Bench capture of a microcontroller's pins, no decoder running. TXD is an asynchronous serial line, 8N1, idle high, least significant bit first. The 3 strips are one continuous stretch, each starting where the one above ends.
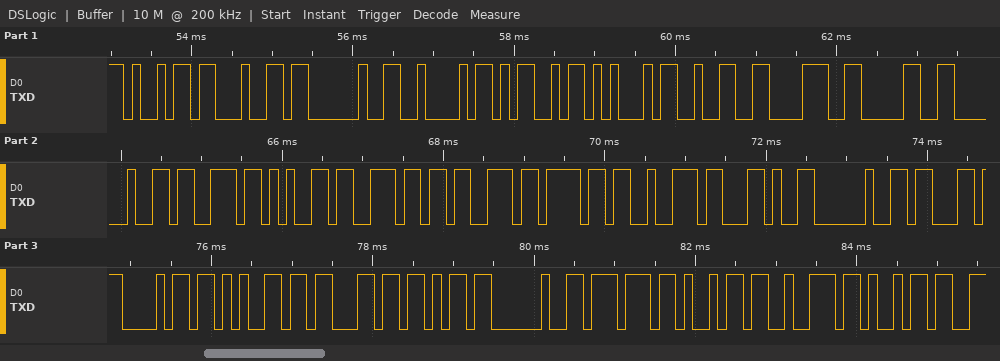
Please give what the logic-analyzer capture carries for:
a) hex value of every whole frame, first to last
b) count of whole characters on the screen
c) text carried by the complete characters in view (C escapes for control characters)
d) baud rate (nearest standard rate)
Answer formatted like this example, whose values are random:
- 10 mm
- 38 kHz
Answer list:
- 69 64 20 42 4D 45 32 38 30 20 73 65 6E 73 6F 72 2C 20 63 68 65 63 6B 20 77 69 72 69
- 28
- "id BME280 sensor, check wiri"
- 9600 baud
